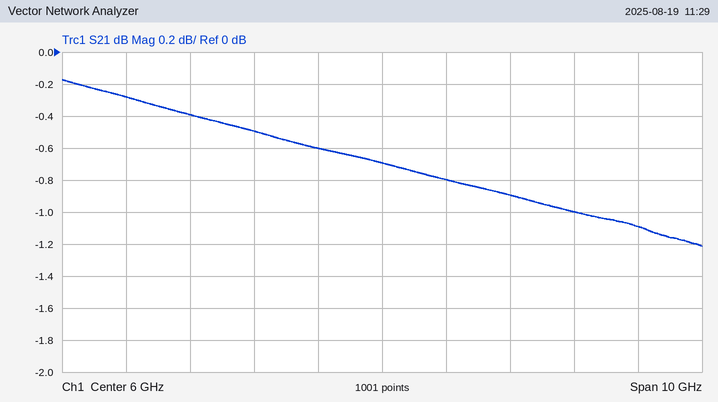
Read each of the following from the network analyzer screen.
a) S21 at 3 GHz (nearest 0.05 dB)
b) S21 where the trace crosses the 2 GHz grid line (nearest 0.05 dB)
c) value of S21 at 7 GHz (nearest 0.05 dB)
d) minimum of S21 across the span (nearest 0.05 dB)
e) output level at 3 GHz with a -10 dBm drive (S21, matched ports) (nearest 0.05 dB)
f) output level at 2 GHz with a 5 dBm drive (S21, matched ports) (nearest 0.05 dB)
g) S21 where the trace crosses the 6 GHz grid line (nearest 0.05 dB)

-0.40 dB
-0.30 dB
-0.80 dB
-1.20 dB
-10.40 dBm
4.70 dBm
-0.70 dB
